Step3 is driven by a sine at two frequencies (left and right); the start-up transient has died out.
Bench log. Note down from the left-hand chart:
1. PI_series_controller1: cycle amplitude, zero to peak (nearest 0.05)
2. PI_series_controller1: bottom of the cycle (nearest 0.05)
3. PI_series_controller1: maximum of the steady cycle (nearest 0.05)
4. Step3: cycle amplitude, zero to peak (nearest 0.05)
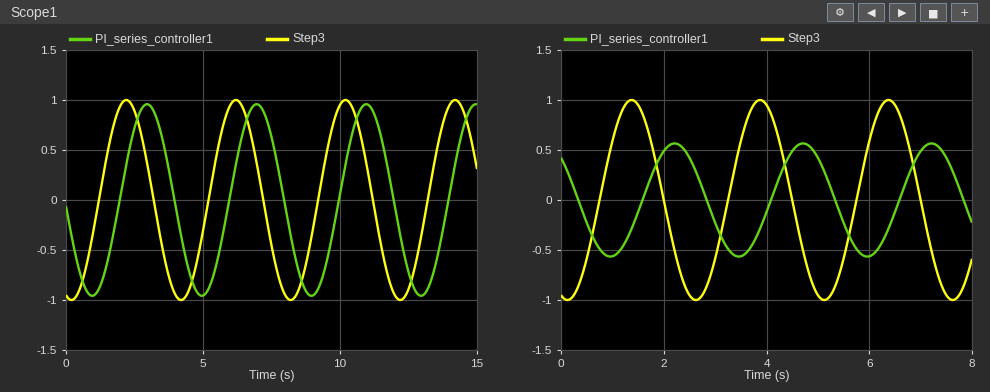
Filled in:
0.95
-0.95
0.95
1.00
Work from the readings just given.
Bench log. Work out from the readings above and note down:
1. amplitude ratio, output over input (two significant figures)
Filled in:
0.95
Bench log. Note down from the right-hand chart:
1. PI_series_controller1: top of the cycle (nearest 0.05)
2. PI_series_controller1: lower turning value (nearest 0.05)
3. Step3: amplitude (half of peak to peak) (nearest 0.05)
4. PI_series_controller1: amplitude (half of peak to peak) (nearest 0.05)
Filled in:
0.55
-0.55
1.00
0.55
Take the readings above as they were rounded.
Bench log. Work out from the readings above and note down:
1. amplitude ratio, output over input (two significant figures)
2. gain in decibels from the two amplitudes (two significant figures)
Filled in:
0.55
-5.2 dB
